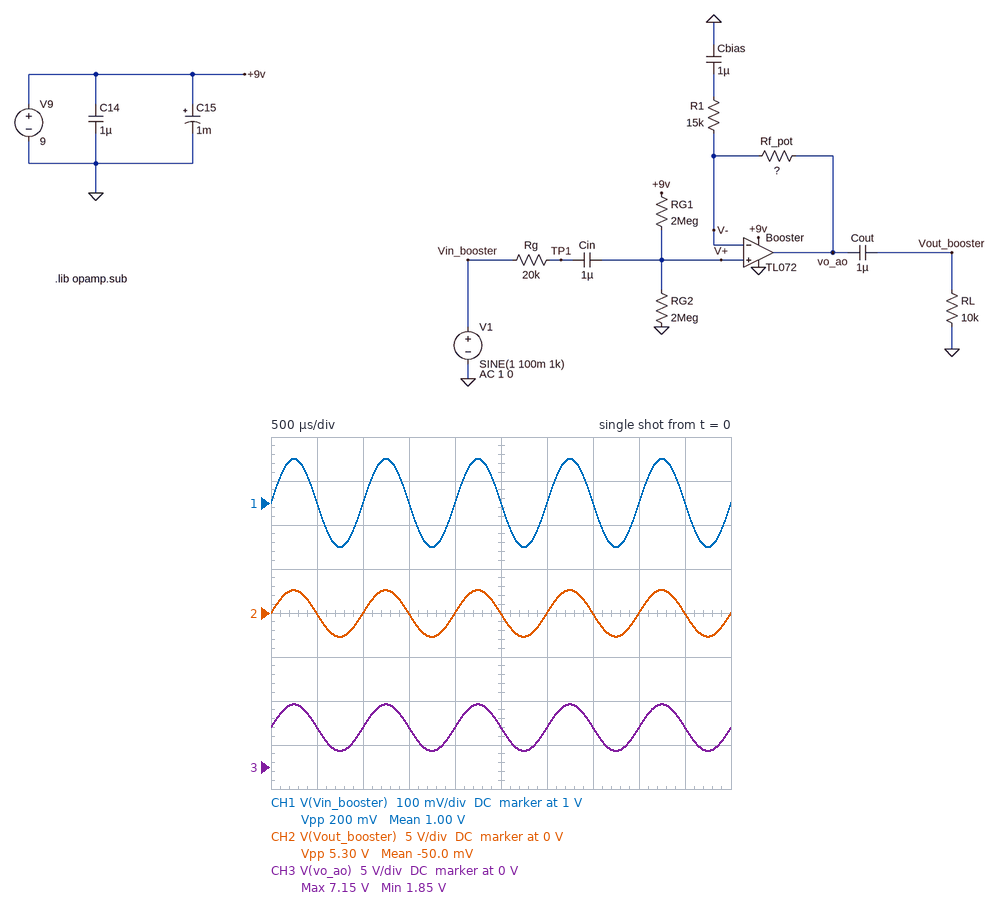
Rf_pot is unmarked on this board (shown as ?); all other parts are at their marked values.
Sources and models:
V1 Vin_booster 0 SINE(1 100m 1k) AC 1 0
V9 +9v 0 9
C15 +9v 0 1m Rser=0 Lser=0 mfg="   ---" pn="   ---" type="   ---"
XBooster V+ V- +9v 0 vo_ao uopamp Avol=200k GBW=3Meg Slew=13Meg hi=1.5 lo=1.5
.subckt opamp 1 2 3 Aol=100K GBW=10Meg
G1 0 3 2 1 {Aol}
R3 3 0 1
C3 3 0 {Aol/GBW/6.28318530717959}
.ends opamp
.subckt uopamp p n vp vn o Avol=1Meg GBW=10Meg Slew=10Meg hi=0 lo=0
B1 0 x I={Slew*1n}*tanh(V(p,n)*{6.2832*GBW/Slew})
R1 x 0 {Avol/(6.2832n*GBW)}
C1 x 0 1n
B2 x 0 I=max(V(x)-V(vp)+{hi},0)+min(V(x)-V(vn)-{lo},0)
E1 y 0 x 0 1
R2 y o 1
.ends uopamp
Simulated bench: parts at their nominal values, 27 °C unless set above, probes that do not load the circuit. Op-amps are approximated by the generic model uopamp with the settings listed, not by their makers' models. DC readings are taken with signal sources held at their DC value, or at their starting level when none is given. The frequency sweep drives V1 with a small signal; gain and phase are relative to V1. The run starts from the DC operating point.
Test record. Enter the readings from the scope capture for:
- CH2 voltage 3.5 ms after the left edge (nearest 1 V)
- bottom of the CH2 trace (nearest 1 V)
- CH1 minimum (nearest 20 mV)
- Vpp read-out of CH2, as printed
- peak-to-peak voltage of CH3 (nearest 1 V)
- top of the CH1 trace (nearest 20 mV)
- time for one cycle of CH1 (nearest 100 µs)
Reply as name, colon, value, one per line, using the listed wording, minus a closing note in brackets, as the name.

CH2 voltage 3.5 ms after the left edge: 0 V
bottom of the CH2 trace: -3 V
CH1 minimum: 900 mV
Vpp read-out of CH2, as printed: 5.30 V
peak-to-peak voltage of CH3: 5 V
top of the CH1 trace: 1.10 V
time for one cycle of CH1: 1.0 ms
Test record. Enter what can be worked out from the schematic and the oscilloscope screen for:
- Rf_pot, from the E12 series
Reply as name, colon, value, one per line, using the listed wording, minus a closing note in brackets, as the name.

Rf_pot, from the E12 series: 390 kΩ
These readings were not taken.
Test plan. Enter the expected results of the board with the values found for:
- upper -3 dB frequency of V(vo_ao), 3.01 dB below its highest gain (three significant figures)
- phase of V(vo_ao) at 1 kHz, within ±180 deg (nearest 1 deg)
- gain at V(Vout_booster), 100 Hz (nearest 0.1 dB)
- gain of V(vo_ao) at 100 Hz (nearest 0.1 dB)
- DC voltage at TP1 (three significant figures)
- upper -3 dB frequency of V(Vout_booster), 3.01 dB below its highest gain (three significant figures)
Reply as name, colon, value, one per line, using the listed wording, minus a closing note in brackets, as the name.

upper -3 dB frequency of V(vo_ao), 3.01 dB below its highest gain: 111 kHz
phase of V(vo_ao) at 1 kHz, within ±180 deg: 0 deg
gain at V(Vout_booster), 100 Hz: 28.3 dB
gain of V(vo_ao) at 100 Hz: 28.4 dB
DC voltage at TP1: 1.00 V
upper -3 dB frequency of V(Vout_booster), 3.01 dB below its highest gain: 111 kHz
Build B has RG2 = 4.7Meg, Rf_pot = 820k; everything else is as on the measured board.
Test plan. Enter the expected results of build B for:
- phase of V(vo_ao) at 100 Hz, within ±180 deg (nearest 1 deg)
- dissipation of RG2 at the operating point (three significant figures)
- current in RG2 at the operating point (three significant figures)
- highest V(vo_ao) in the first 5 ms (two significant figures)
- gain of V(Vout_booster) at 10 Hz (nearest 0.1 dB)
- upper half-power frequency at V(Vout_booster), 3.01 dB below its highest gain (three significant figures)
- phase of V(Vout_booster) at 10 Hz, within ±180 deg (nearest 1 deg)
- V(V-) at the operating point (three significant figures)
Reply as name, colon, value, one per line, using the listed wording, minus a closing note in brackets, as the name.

phase of V(vo_ao) at 100 Hz, within ±180 deg: 6 deg
dissipation of RG2 at the operating point: 8.48 µW
current in RG2 at the operating point: 1.34 µA
highest V(vo_ao) in the first 5 ms: 7.5 V
gain of V(Vout_booster) at 10 Hz: 26.0 dB
upper half-power frequency at V(Vout_booster), 3.01 dB below its highest gain: 53.9 kHz
phase of V(Vout_booster) at 10 Hz, within ±180 deg: 104 deg
V(V-) at the operating point: 6.31 V
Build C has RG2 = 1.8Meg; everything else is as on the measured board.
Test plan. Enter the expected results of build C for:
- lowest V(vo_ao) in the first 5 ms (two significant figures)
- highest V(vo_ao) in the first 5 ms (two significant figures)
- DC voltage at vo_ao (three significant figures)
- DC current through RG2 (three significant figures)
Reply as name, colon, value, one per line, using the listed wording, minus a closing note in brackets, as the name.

lowest V(vo_ao) in the first 5 ms: 1.6 V
highest V(vo_ao) in the first 5 ms: 6.9 V
DC voltage at vo_ao: 4.26 V
DC current through RG2: 2.37 µA
